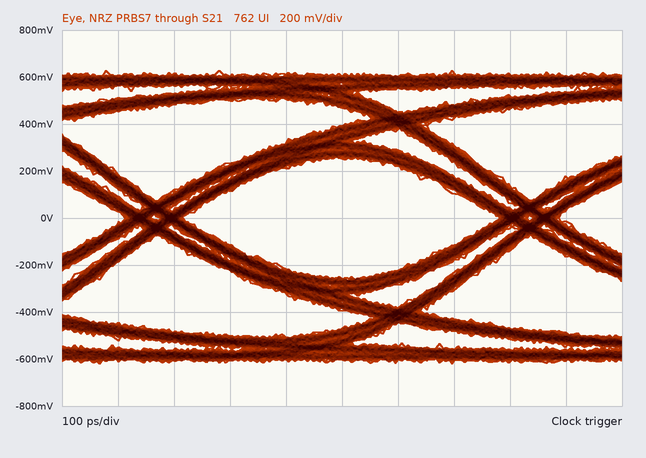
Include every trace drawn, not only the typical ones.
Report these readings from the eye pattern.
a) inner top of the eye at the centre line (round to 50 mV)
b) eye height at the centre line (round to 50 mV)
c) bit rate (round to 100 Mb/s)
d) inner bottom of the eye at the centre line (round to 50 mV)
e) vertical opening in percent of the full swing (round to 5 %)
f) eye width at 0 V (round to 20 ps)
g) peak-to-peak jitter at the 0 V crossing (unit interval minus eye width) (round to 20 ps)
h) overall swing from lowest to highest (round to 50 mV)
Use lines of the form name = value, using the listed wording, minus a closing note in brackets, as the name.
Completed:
inner top of the eye at the centre line = 250 mV
eye height at the centre line = 500 mV
bit rate = 1.5 Gb/s
inner bottom of the eye at the centre line = -250 mV
vertical opening in percent of the full swing = 40 %
eye width at 0 V = 560 ps
peak-to-peak jitter at the 0 V crossing (unit interval minus eye width) = 100 ps
overall swing from lowest to highest = 1.25 V
